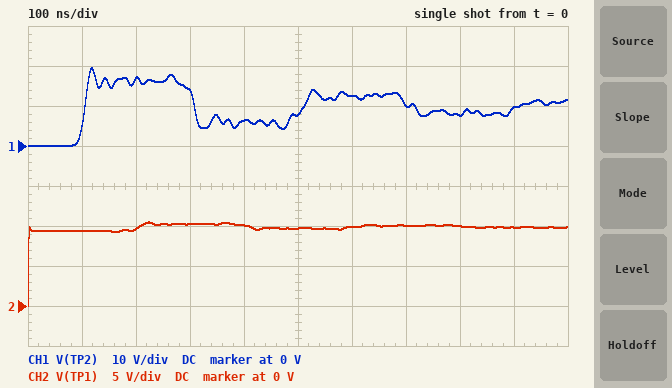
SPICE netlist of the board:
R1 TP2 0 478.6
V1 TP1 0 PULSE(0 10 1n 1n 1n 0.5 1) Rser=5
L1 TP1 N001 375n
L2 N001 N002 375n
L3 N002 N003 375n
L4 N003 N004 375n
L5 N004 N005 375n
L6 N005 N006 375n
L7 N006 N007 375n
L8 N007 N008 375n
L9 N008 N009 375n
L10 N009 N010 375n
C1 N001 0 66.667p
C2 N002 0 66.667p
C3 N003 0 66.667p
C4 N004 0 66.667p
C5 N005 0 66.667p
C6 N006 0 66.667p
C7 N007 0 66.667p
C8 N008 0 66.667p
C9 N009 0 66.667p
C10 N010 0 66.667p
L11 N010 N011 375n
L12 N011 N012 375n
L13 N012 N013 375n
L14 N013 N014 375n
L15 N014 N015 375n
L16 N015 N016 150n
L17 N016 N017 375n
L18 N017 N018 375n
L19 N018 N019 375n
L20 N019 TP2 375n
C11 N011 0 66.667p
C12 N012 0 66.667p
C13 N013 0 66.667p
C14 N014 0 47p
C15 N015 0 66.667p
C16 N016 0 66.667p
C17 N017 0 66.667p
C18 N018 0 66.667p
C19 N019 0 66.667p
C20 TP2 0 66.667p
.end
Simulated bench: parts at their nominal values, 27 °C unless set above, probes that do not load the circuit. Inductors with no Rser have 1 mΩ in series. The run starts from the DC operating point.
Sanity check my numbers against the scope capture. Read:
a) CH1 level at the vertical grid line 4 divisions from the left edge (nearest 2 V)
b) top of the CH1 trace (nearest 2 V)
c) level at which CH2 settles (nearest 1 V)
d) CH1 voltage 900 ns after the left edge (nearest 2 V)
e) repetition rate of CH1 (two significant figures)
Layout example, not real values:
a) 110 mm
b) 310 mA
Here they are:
a) 6 V
b) 20 V
c) 10 V
d) 10 V
e) 2.5 MHz
